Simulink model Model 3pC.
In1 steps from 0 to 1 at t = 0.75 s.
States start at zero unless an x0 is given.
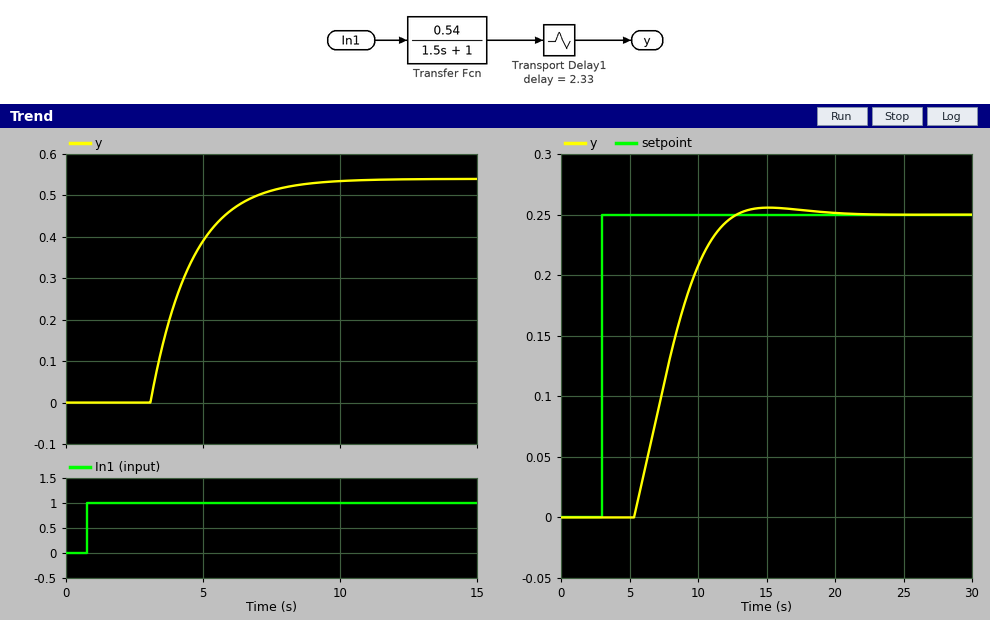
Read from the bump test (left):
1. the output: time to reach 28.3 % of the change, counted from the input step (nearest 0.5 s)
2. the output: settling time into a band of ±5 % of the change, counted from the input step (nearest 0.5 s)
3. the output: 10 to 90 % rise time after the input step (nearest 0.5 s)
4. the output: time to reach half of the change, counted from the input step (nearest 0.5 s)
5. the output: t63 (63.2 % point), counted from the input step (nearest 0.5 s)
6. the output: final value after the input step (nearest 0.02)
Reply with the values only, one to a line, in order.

3.0 s
7.0 s
3.5 s
3.5 s
4.0 s
0.54
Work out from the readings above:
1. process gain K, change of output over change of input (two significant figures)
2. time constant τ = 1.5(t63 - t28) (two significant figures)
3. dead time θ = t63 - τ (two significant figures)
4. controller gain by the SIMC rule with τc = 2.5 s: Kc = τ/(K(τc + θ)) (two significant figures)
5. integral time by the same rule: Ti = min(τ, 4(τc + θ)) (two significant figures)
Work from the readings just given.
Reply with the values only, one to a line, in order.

0.54
1.5 s
2.5 s
0.56
1.5 s
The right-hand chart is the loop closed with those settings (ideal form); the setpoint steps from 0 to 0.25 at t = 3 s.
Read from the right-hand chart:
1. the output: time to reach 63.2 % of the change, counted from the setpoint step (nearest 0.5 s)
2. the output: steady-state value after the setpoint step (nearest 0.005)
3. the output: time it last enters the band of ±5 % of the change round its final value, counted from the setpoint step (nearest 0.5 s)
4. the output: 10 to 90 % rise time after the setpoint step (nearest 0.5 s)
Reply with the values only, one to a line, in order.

5.5 s
0.250
8.5 s
5.0 s
